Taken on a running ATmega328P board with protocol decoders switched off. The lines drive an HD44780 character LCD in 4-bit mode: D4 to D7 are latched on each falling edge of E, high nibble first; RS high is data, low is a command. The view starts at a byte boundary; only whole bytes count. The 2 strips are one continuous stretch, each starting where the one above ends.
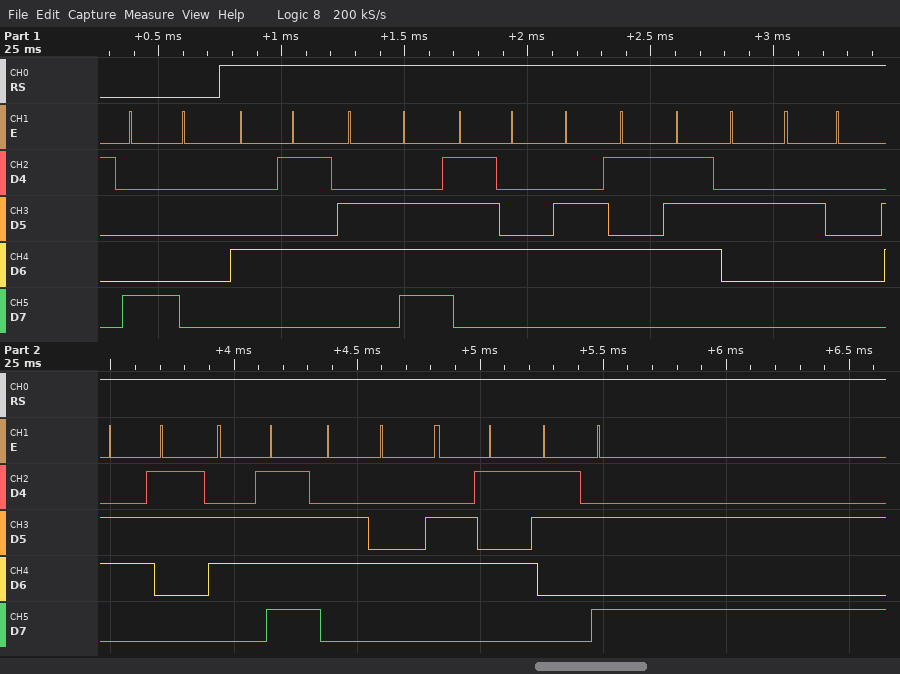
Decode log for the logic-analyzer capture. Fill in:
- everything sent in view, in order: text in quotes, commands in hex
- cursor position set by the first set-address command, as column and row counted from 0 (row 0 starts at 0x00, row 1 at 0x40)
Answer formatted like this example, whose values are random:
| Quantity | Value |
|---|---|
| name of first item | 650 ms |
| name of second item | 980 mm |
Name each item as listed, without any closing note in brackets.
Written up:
| Quantity | Value |
|---|---|
| everything sent in view, in order: text in quotes, commands in hex | 0x80 "Enter code:" |
| cursor position set by the first set-address command, as column and row counted from 0 | column 0, row 0 |
